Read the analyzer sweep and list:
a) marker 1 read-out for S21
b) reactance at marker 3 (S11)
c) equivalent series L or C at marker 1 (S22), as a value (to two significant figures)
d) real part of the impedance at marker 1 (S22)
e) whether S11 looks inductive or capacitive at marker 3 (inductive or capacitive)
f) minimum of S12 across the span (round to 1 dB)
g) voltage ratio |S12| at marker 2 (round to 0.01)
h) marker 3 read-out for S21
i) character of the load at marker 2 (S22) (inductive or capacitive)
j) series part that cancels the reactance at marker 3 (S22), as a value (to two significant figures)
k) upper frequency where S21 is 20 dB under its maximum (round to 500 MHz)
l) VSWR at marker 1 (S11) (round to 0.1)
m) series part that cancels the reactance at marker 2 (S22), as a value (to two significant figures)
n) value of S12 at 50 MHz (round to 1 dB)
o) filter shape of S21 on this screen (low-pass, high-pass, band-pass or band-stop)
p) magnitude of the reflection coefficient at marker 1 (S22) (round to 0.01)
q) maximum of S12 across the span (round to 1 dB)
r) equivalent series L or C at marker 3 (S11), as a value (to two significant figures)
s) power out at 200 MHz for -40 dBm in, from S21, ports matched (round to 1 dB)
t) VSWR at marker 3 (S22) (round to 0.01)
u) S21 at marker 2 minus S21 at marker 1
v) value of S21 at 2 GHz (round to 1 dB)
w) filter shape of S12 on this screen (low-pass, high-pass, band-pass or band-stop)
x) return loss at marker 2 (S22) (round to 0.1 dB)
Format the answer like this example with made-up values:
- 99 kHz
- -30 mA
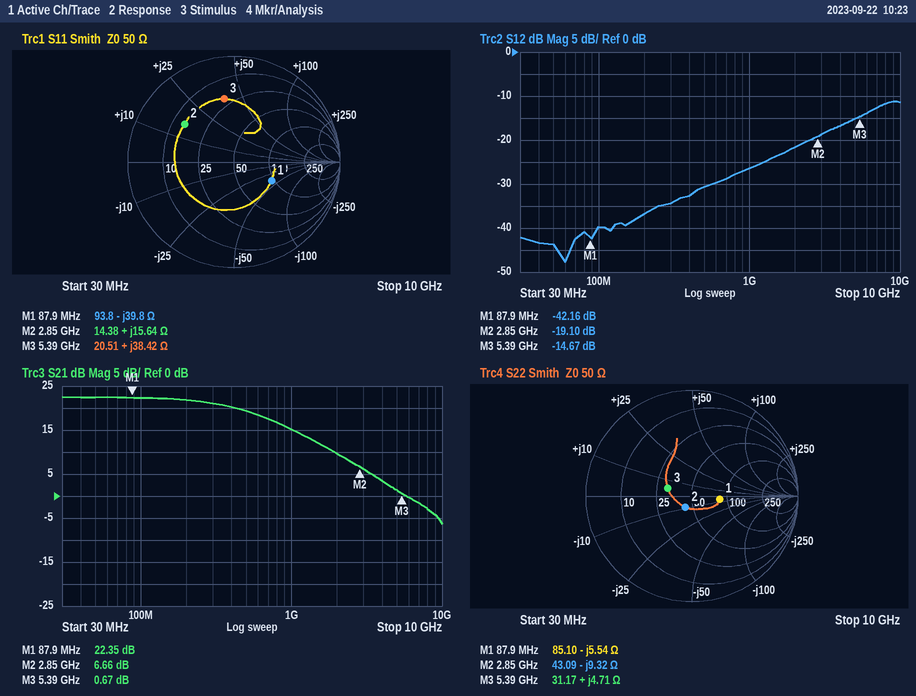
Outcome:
- 22.35 dB
- +38.42 Ω
- 330 pF
- 85.10 Ω
- inductive
- -48 dB
- 0.11
- 0.67 dB
- capacitive
- 6.3 pF
- 4.5 GHz
- 2.3
- 520 pH
- -44 dB
- low-pass
- 0.26
- -11 dB
- 1.1 nH
- -18 dBm
- 1.63
- -15.69 dB
- 10 dB
- high-pass
- 18.1 dB
